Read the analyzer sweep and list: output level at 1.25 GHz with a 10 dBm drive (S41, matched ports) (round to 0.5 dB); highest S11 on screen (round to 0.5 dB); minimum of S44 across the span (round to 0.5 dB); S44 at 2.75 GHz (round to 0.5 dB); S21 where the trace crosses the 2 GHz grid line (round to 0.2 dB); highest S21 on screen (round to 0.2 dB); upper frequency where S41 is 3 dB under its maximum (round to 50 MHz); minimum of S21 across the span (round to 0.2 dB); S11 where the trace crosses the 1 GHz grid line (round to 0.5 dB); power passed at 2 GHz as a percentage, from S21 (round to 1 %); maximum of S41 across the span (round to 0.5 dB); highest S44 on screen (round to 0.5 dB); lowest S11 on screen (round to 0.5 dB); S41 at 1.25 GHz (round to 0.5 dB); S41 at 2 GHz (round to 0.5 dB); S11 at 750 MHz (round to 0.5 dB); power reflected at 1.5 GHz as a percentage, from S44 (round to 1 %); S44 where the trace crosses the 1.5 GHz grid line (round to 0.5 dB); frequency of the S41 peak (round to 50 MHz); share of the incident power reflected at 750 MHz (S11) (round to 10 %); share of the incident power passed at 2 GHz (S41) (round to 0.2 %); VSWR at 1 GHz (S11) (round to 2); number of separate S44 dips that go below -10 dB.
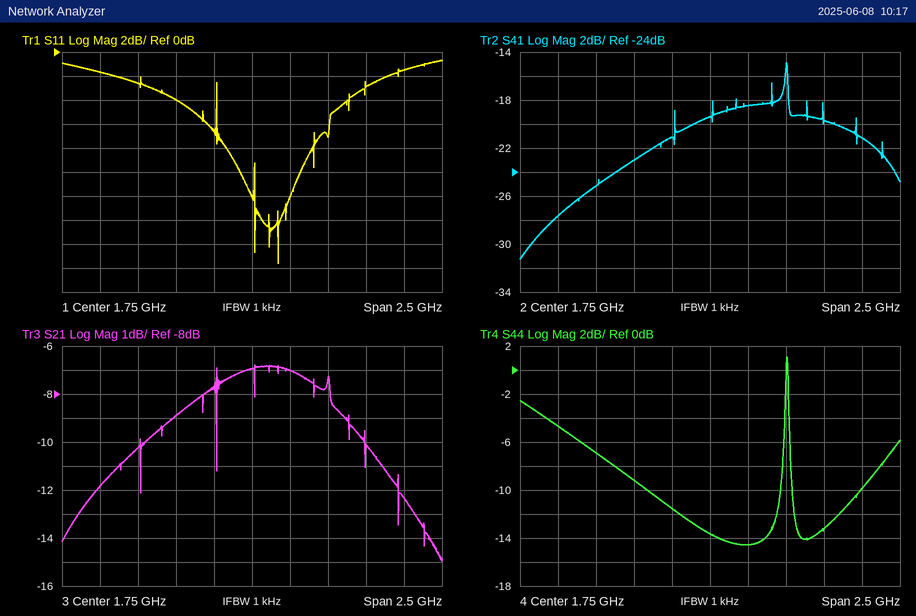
-13.0 dBm
-0.5 dB
-14.5 dB
-10.0 dB
-7.0 dB
-6.8 dB
2.25 GHz
-15.0 dB
-2.5 dB
20 %
-15.0 dB
1.0 dB
-17.5 dB
-23.0 dB
-18.5 dB
-1.5 dB
7 %
-11.5 dB
2.25 GHz
70 %
1.4 %
6
2
